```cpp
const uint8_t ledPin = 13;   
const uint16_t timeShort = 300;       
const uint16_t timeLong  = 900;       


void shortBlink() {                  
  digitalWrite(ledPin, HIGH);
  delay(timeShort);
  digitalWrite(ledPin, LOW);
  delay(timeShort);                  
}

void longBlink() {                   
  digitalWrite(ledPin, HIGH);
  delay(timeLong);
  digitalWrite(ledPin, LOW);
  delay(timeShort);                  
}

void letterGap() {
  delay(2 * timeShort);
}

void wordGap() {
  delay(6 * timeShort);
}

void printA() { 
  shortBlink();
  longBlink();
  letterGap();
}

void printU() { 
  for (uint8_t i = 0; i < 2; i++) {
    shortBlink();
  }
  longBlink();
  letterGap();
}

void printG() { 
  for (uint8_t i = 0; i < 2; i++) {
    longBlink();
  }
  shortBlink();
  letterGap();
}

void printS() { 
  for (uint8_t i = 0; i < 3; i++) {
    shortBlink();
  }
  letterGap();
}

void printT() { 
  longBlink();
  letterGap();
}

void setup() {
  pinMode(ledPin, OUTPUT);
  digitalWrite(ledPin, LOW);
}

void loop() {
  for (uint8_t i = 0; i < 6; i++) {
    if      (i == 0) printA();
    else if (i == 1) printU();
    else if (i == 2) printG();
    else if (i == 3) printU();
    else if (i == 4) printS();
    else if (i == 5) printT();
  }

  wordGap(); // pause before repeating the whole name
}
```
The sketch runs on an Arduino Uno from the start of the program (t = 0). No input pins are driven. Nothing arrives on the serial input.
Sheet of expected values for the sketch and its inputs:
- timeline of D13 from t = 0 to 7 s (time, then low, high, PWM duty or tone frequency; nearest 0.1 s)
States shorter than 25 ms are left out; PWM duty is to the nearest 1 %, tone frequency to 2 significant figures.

0 s high; 0.3 s low; 0.6 s high; 1.5 s low; 2.4 s high; 2.7 s low; 3 s high; 3.3 s low; 3.6 s high; 4.5 s low; 5.4 s high; 6.3 s low; 6.6 s high
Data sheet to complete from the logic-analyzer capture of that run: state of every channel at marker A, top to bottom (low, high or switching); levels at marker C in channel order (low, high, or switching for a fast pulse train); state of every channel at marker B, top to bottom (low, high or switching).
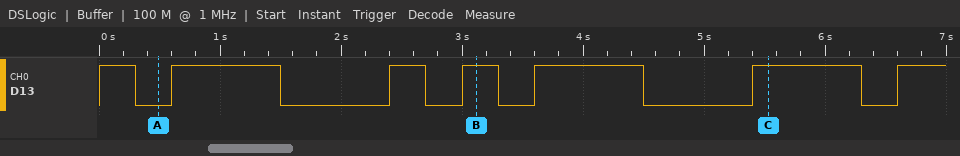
D13 low
D13 high
D13 high
